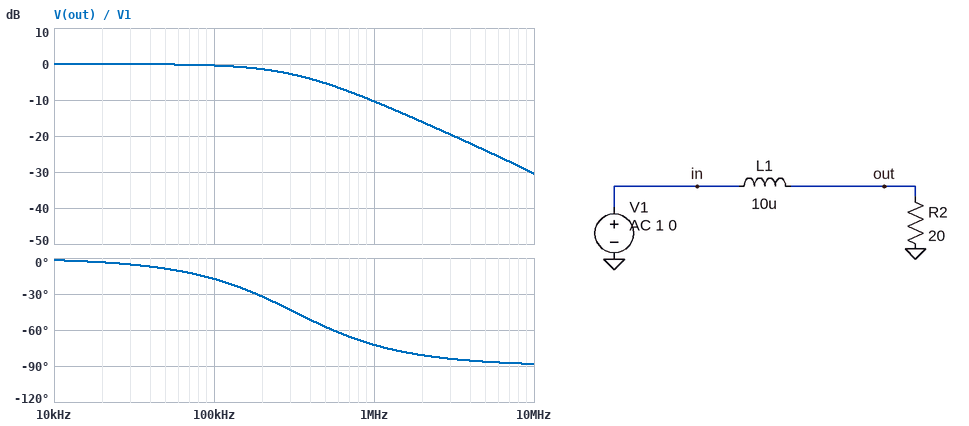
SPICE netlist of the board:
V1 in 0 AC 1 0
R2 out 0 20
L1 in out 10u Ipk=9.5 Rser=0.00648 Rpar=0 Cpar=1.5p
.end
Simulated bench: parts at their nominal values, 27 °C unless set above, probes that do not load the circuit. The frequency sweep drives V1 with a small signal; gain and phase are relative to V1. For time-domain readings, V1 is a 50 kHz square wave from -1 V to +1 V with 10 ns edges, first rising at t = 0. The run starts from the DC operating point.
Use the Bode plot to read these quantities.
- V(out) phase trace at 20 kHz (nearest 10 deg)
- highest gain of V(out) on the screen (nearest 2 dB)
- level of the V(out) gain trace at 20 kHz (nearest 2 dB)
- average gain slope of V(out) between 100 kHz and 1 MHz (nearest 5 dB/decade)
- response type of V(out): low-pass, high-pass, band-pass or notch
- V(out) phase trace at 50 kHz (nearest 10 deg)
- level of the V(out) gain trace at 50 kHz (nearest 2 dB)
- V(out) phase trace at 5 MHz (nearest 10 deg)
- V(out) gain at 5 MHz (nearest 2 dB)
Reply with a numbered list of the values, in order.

1. 0 deg
2. 0 dB
3. 0 dB
4. -10 dB/decade
5. low-pass
6. -10 deg
7. 0 dB
8. -90 deg
9. -24 dB
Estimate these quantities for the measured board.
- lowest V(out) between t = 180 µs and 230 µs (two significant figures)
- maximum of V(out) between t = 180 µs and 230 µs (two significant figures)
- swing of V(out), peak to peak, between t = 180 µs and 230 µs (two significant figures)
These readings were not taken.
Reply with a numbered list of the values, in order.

1. -1.0 V
2. 1.0 V
3. 2.0 V
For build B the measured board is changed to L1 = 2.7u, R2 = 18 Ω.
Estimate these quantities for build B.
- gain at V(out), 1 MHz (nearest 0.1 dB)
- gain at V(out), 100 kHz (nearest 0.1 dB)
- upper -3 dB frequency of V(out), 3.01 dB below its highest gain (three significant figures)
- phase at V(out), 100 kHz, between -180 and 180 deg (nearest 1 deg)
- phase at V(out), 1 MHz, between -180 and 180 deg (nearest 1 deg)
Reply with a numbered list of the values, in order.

1. -2.8 dB
2. 0 dB
3. 1.06 MHz
4. -5 deg
5. -43 deg
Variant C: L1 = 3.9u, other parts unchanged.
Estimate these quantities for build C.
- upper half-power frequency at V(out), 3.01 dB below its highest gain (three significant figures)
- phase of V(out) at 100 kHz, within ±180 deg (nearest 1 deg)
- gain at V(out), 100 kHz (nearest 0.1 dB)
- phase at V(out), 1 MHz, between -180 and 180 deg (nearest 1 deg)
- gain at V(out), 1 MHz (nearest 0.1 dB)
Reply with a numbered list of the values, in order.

1. 816 kHz
2. -7 deg
3. -0.1 dB
4. -51 deg
5. -4.0 dB
